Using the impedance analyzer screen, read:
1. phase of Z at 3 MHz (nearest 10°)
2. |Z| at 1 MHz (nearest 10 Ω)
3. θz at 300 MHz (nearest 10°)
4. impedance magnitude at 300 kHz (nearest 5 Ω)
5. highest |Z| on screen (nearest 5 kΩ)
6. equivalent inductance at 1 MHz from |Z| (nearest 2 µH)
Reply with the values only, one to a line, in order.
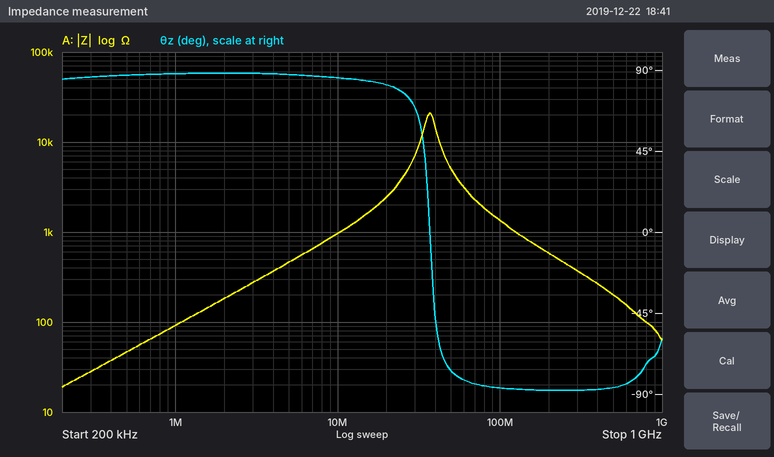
90°
90 Ω
-90°
30 Ω
20 kΩ
14 µH
